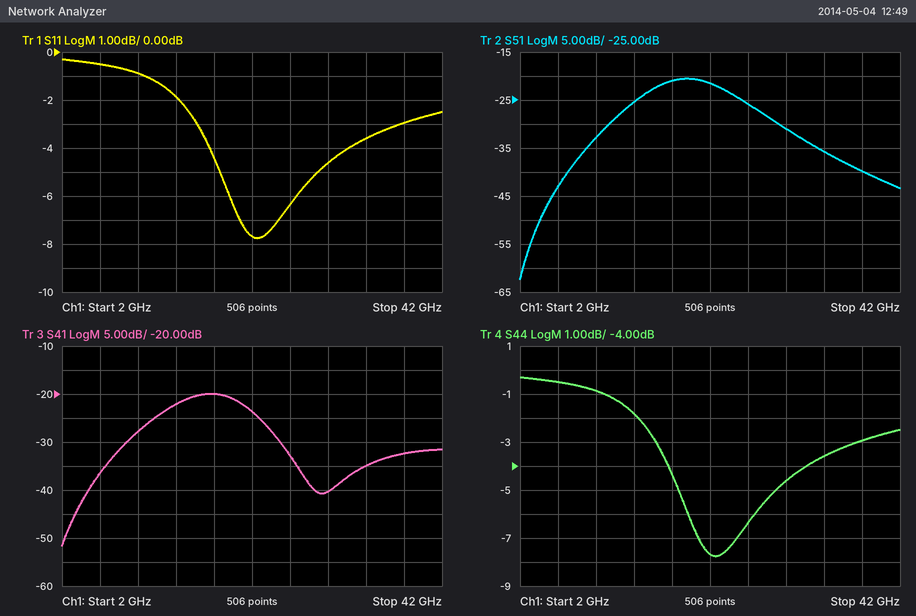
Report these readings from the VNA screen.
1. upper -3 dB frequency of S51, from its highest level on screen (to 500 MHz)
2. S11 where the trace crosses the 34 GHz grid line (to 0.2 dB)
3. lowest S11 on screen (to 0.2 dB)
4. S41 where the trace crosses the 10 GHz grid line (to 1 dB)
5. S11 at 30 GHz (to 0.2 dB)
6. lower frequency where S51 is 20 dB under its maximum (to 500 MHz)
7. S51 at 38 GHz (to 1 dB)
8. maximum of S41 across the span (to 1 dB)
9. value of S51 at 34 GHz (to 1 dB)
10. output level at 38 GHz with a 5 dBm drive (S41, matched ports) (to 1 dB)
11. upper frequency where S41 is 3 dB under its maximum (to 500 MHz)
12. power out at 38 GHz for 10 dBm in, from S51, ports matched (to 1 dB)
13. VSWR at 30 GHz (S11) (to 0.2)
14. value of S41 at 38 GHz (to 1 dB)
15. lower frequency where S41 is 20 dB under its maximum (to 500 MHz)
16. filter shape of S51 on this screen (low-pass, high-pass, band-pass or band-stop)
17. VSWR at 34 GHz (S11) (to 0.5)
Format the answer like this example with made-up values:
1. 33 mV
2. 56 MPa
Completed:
1. 24.0 GHz
2. -3.6 dB
3. -7.8 dB
4. -28 dB
5. -4.6 dB
6. 7.0 GHz
7. -40 dB
8. -20 dB
9. -36 dB
10. -27 dBm
11. 21.5 GHz
12. -30 dBm
13. 3.8
14. -32 dB
15. 5.0 GHz
16. band-pass
17. 5.0
